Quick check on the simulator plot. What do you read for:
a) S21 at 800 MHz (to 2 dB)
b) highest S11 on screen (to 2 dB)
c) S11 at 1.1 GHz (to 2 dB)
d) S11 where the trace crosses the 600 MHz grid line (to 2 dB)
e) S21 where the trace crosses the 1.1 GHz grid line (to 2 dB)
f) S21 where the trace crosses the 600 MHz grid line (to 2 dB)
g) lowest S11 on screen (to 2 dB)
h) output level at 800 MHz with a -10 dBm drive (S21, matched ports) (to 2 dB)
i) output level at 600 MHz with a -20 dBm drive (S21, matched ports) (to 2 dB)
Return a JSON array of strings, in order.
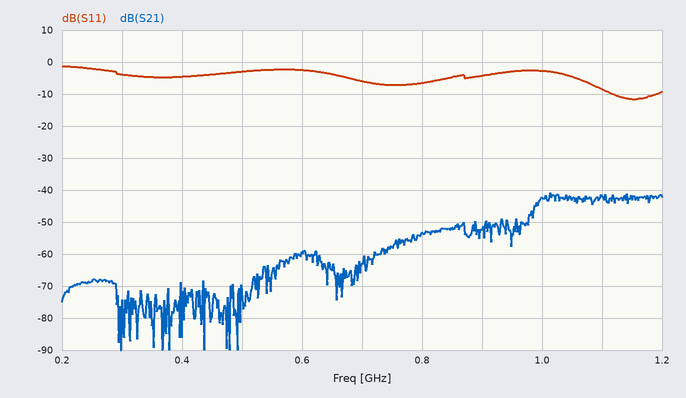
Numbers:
["-54 dB", "-2 dB", "-8 dB", "-2 dB", "-42 dB", "-60 dB", "-12 dB", "-64 dBm", "-80 dBm"]
